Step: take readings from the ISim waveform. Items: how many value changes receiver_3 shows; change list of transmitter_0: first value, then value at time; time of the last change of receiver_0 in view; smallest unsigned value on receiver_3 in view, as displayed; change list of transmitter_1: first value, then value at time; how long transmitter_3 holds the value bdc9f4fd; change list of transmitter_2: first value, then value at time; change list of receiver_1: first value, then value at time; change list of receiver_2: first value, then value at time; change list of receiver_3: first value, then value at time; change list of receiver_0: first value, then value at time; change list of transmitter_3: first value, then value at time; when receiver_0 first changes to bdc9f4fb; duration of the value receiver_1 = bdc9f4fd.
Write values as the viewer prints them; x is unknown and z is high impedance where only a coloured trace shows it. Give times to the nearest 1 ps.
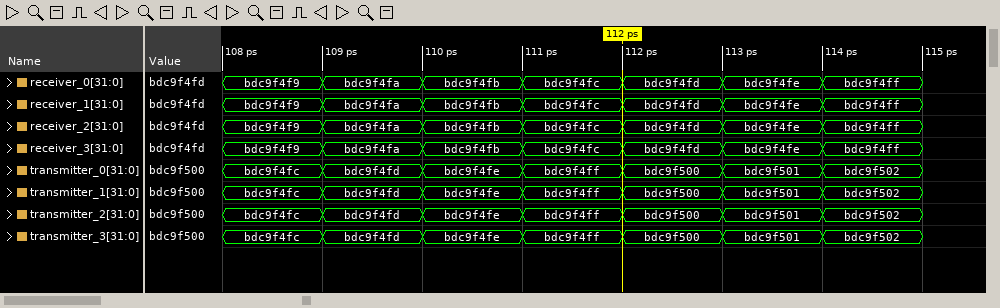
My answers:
6
bdc9f4fc, bdc9f4fd at 109 ps, bdc9f4fe at 110 ps, bdc9f4ff at 111 ps, bdc9f500 at 112 ps, bdc9f501 at 113 ps, bdc9f502 at 114 ps
114 ps
bdc9f4f9
bdc9f4fc, bdc9f4fd at 109 ps, bdc9f4fe at 110 ps, bdc9f4ff at 111 ps, bdc9f500 at 112 ps, bdc9f501 at 113 ps, bdc9f502 at 114 ps
1 ps
bdc9f4fc, bdc9f4fd at 109 ps, bdc9f4fe at 110 ps, bdc9f4ff at 111 ps, bdc9f500 at 112 ps, bdc9f501 at 113 ps, bdc9f502 at 114 ps
bdc9f4f9, bdc9f4fa at 109 ps, bdc9f4fb at 110 ps, bdc9f4fc at 111 ps, bdc9f4fd at 112 ps, bdc9f4fe at 113 ps, bdc9f4ff at 114 ps
bdc9f4f9, bdc9f4fa at 109 ps, bdc9f4fb at 110 ps, bdc9f4fc at 111 ps, bdc9f4fd at 112 ps, bdc9f4fe at 113 ps, bdc9f4ff at 114 ps
bdc9f4f9, bdc9f4fa at 109 ps, bdc9f4fb at 110 ps, bdc9f4fc at 111 ps, bdc9f4fd at 112 ps, bdc9f4fe at 113 ps, bdc9f4ff at 114 ps
bdc9f4f9, bdc9f4fa at 109 ps, bdc9f4fb at 110 ps, bdc9f4fc at 111 ps, bdc9f4fd at 112 ps, bdc9f4fe at 113 ps, bdc9f4ff at 114 ps
bdc9f4fc, bdc9f4fd at 109 ps, bdc9f4fe at 110 ps, bdc9f4ff at 111 ps, bdc9f500 at 112 ps, bdc9f501 at 113 ps, bdc9f502 at 114 ps
110 ps
1 ps
